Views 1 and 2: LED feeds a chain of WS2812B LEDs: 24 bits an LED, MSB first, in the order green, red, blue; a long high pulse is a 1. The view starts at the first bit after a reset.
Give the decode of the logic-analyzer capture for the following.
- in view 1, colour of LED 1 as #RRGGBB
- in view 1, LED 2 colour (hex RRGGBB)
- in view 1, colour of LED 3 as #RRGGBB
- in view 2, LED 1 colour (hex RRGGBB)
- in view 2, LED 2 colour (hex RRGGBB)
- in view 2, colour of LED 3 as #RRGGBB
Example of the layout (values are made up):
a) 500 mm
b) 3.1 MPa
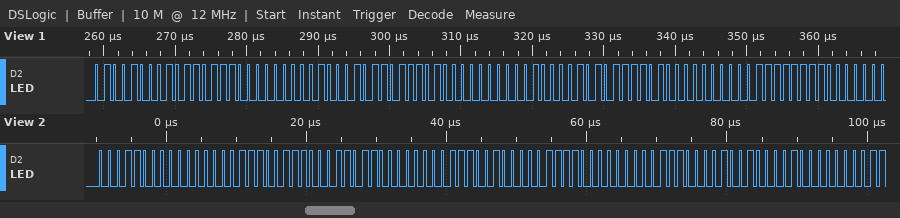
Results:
a) #B74800
b) #BA4500
c) #BD4200
d) #0018E7
e) #001BE4
f) #001EE1
